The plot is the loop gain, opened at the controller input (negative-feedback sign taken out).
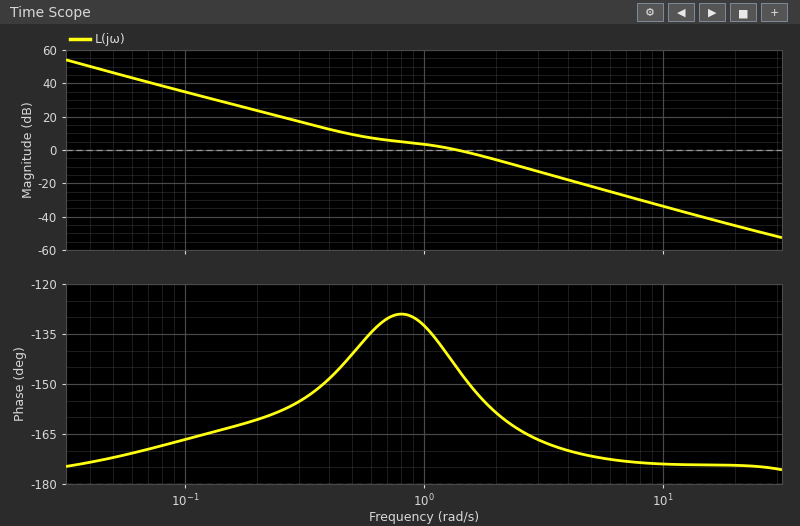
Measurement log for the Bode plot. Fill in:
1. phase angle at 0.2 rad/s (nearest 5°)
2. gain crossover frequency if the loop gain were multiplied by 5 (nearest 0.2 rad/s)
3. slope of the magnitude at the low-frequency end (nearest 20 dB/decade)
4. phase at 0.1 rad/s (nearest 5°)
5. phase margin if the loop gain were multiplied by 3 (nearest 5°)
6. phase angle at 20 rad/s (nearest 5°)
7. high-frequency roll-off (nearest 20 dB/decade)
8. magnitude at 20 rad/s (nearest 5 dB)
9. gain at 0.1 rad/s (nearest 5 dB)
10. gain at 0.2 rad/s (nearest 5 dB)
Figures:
-160°
3.2 rad/s
-40 dB/decade
-165°
15°
-175°
-40 dB/decade
-45 dB
35 dB
25 dB
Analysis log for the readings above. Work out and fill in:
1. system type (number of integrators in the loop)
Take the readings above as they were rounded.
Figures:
2
